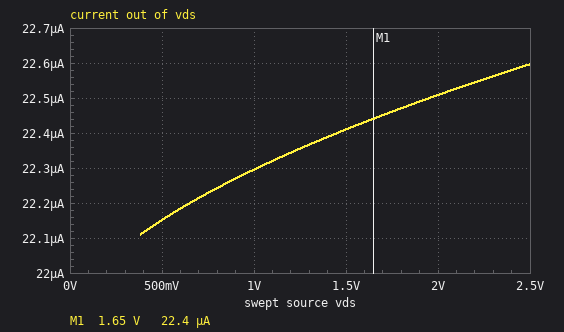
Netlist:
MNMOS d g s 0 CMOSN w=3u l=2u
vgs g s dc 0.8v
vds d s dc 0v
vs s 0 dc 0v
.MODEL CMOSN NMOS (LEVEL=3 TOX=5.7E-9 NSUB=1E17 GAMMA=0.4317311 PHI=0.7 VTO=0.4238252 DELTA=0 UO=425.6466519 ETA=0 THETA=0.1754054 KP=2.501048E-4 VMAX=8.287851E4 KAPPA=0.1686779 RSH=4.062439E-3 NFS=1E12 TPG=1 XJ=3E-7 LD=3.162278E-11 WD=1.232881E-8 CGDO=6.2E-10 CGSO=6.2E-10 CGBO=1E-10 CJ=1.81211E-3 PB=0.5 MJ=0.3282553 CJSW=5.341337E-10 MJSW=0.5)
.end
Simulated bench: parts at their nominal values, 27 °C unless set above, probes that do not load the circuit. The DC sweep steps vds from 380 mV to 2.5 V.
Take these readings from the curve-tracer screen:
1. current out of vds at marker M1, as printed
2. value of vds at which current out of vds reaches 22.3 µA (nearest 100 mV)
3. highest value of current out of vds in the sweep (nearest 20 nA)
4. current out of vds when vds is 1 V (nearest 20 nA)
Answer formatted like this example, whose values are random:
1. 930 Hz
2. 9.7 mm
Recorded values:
1. 22.4 µA
2. 1.0 V
3. 22.60 µA
4. 22.30 µA
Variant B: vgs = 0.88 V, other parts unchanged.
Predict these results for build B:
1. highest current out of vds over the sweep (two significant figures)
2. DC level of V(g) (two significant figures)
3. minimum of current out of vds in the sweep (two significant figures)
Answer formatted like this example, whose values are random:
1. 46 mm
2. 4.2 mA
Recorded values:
1. 32 µA
2. 880 mV
3. 31 µA
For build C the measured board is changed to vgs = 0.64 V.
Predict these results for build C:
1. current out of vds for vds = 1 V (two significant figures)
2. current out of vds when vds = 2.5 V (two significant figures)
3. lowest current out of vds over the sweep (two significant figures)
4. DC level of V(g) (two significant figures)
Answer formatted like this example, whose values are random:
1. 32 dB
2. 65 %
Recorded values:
1. 8.3 µA
2. 8.4 µA
3. 8.2 µA
4. 640 mV
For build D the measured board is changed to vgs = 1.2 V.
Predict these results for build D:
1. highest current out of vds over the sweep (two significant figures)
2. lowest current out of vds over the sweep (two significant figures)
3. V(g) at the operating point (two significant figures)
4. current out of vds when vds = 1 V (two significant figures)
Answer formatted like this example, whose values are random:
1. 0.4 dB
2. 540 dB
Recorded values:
1. 81 µA
2. 66 µA
3. 1.2 V
4. 80 µA
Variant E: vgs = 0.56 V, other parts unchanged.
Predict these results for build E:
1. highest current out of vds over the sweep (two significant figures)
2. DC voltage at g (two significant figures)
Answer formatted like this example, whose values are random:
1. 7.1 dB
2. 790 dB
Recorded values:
1. 3.7 µA
2. 560 mV
